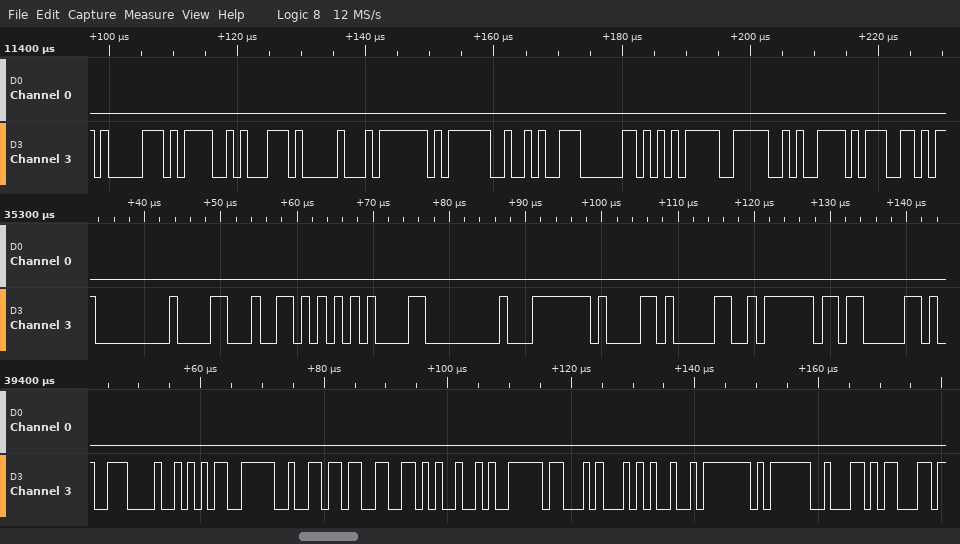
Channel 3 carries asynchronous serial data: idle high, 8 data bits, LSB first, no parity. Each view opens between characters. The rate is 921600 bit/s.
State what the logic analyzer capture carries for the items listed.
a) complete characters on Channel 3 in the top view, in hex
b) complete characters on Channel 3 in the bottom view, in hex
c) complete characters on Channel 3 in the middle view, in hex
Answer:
C1, 3D, 71, 10, 7F, 3F, CA, 60, F5, 3E, 79, 67
0E, AA, 3E, B6, 66, 49, BE, 14, 25, 7F, 3F, AC
00, 18, 56, 85, 00, FC, 61, 30, BF, 83
